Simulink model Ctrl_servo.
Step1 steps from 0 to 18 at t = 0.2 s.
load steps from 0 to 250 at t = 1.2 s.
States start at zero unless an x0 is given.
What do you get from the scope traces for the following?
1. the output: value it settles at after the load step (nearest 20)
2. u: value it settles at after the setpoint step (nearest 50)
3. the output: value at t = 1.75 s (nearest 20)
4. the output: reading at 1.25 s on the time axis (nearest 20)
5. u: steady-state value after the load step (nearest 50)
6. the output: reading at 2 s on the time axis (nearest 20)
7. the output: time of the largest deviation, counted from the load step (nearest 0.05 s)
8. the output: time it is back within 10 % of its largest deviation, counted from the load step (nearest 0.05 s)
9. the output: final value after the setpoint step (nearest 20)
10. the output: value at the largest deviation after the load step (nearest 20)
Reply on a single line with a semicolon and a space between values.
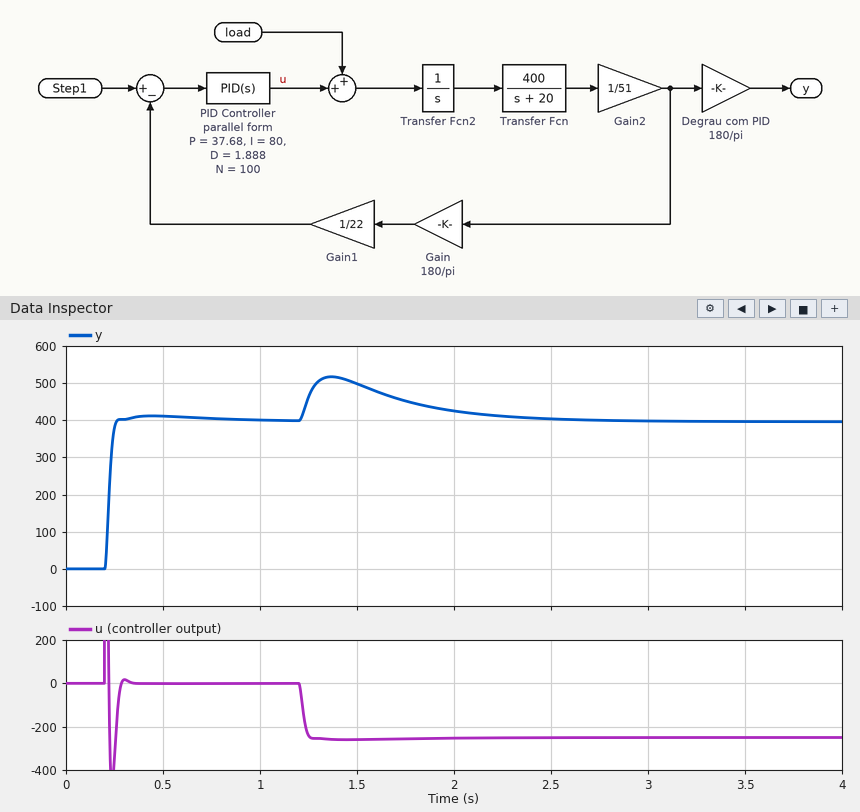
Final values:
400; 0; 460; 460; -250; 420; 0.15 s; 1.15 s; 400; 520
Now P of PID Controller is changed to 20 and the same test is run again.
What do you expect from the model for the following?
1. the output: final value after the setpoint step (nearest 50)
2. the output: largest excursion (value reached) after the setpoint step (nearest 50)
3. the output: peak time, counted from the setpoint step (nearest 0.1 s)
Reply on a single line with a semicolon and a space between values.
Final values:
400; 450; 0.4 s
